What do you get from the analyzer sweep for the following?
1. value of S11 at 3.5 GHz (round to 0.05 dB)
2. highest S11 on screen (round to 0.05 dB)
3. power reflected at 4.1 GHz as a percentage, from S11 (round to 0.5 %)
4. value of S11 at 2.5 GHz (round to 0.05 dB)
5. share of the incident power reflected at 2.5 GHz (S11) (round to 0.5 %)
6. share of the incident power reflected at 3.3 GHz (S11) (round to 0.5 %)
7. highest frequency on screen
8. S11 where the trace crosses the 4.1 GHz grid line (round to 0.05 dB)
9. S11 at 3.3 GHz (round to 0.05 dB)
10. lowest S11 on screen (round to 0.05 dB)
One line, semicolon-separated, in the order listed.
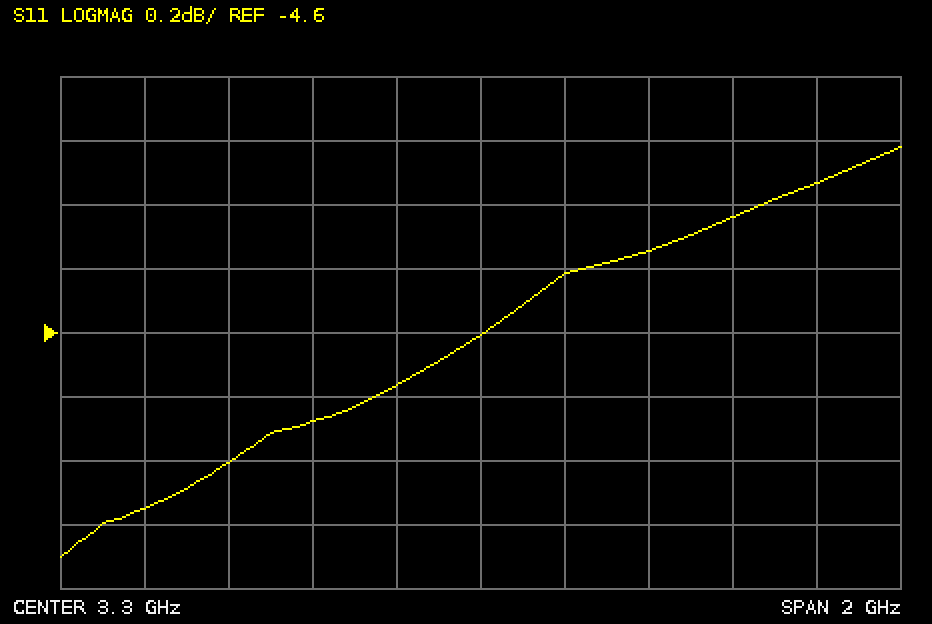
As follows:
-4.40 dB; -4.00 dB; 38.5 %; -5.15 dB; 30.5 %; 34.5 %; 4.3 GHz; -4.15 dB; -4.60 dB; -5.30 dB
